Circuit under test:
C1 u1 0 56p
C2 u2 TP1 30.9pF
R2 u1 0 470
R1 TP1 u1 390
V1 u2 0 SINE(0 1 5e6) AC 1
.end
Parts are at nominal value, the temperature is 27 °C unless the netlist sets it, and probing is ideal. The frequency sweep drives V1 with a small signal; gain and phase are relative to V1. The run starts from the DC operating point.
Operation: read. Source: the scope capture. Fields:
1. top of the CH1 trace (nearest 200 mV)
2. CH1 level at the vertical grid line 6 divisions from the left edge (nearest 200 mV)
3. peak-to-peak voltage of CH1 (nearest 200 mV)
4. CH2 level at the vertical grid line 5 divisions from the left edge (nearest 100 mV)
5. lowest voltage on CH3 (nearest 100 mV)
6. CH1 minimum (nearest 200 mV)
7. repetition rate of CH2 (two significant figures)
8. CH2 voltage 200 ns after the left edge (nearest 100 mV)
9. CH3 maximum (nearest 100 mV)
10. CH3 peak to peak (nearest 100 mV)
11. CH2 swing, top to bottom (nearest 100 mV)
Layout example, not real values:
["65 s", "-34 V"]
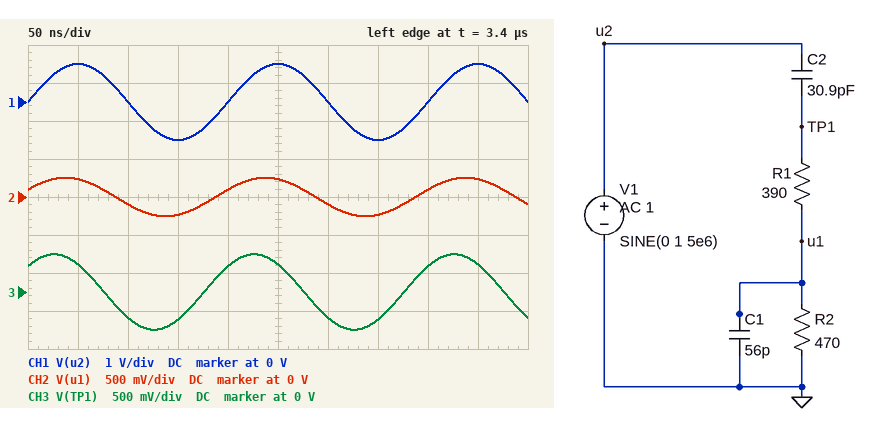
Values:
["1.0 V", "0 V", "2.0 V", "200 mV", "-500 mV", "-1.0 V", "5.0 MHz", "100 mV", "500 mV", "1.0 V", "500 mV"]
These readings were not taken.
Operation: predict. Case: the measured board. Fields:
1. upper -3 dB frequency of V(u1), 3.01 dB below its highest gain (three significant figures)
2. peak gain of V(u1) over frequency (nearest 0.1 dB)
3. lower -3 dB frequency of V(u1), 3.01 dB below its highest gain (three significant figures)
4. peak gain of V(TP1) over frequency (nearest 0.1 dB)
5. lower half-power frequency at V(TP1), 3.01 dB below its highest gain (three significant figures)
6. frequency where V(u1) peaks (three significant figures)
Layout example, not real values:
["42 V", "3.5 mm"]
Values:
["29.3 MHz", "-11.2 dB", "2.73 MHz", "0 dB", "14.8 MHz", "8.94 MHz"]
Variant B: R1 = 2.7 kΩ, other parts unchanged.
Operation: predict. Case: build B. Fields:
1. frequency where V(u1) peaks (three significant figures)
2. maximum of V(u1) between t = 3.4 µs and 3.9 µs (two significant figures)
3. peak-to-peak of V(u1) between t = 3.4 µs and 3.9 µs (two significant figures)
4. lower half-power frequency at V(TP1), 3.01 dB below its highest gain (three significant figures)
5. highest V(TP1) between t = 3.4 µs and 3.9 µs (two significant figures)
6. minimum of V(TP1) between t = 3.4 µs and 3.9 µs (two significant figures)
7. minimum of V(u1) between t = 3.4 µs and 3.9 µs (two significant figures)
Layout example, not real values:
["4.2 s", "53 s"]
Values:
["3.40 MHz", "110 mV", "220 mV", "1.71 MHz", "920 mV", "-920 mV", "-110 mV"]
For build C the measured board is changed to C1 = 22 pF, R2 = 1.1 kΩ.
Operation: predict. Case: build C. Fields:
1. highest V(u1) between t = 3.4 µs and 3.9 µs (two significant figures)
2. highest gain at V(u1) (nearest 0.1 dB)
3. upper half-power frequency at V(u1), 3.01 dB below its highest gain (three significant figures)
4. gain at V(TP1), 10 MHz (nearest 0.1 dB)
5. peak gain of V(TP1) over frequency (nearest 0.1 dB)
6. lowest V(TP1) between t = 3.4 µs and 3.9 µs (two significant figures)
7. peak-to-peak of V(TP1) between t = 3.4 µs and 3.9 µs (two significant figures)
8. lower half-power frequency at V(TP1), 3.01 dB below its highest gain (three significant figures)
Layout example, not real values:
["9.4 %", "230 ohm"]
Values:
["460 mV", "-6.3 dB", "40.5 MHz", "-3.0 dB", "0 dB", "-640 mV", "1.3 V", "10.2 MHz"]
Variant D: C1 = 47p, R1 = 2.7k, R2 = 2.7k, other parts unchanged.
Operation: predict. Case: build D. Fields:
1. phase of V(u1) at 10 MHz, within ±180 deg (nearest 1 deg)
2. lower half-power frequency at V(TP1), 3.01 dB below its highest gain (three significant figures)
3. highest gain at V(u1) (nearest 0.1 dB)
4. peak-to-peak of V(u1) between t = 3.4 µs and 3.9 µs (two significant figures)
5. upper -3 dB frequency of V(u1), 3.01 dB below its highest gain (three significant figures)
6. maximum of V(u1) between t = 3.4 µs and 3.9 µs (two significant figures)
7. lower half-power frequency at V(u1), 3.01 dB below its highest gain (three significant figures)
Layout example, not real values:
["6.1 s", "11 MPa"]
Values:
["-66 deg", "1.92 MHz", "-10.9 dB", "400 mV", "4.90 MHz", "200 mV", "488 kHz"]
